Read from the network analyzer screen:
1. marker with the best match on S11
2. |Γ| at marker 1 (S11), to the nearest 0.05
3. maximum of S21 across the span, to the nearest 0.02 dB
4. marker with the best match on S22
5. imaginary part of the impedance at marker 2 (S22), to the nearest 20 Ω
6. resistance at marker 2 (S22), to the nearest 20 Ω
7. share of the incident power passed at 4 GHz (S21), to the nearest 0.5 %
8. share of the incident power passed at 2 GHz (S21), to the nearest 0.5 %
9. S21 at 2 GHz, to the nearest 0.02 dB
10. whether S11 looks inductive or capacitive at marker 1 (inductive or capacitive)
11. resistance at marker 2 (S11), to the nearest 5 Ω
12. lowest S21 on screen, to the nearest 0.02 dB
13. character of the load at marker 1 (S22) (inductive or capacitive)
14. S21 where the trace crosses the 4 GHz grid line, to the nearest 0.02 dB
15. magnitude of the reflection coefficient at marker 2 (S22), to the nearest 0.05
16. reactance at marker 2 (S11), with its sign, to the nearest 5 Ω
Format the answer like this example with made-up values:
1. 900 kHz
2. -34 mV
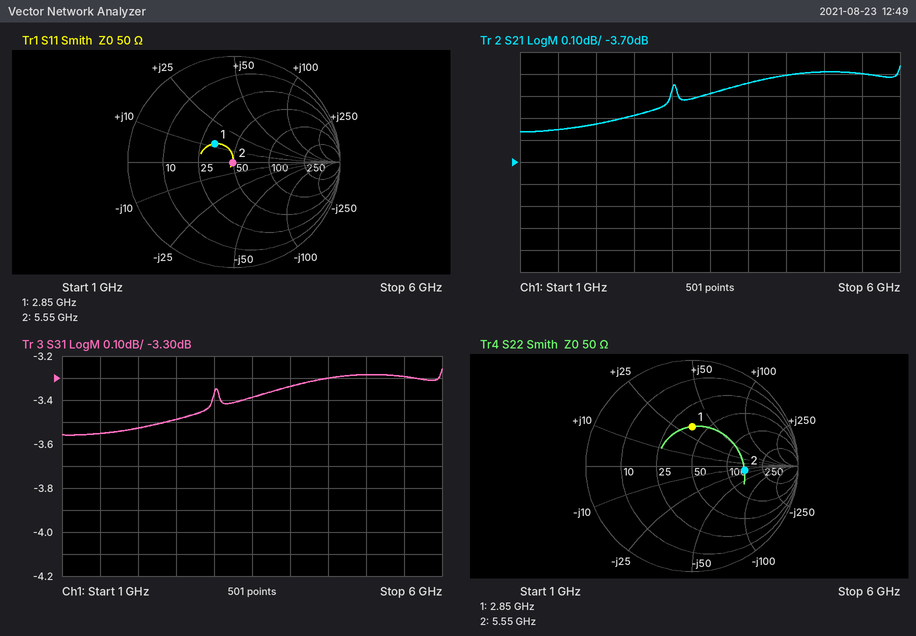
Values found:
1. marker 2
2. 0.25
3. -3.26 dB
4. marker 1
5. -20 Ω
6. 140 Ω
7. 46.5 %
8. 44.5 %
9. -3.52 dB
10. inductive
11. 50 Ω
12. -3.56 dB
13. inductive
14. -3.34 dB
15. 0.50
16. 0 Ω
